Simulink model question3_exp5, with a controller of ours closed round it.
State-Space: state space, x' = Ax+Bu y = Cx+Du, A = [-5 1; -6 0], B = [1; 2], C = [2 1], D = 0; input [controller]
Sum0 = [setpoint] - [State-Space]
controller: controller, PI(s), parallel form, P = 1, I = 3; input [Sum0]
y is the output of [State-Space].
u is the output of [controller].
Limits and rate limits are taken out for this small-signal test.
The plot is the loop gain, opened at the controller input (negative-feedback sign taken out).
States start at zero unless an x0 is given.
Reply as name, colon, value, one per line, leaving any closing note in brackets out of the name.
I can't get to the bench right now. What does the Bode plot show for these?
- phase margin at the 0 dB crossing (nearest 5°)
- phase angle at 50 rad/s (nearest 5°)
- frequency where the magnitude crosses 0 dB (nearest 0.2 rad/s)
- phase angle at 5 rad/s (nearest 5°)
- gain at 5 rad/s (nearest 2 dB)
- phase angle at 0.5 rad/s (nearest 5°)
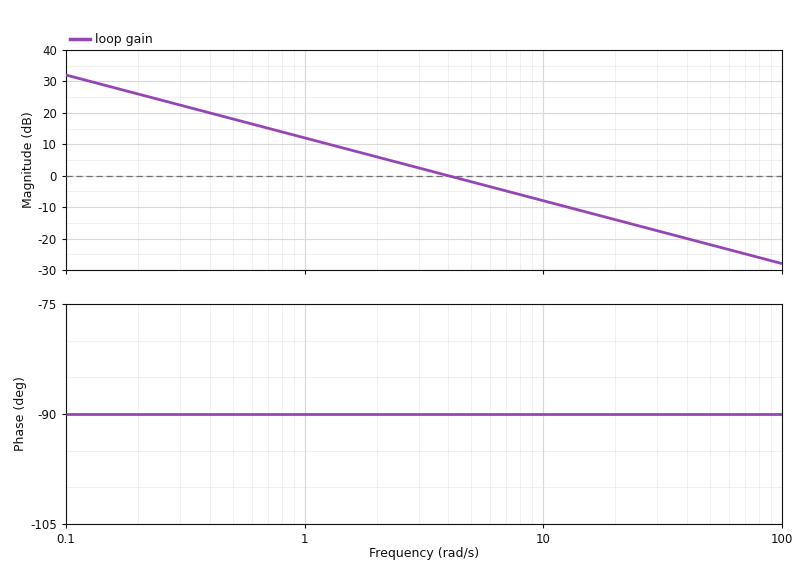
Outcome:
phase margin at the 0 dB crossing: 90°
phase angle at 50 rad/s: -90°
frequency where the magnitude crosses 0 dB: 4.0 rad/s
phase angle at 5 rad/s: -90°
gain at 5 rad/s: -2 dB
phase angle at 0.5 rad/s: -90°
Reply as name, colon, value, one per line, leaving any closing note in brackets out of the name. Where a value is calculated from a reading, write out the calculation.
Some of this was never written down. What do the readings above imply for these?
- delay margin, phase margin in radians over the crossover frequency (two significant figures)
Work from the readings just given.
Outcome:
delay margin, phase margin in radians over the crossover frequency: 90 × π / 180 / 4 = 0.39 s
